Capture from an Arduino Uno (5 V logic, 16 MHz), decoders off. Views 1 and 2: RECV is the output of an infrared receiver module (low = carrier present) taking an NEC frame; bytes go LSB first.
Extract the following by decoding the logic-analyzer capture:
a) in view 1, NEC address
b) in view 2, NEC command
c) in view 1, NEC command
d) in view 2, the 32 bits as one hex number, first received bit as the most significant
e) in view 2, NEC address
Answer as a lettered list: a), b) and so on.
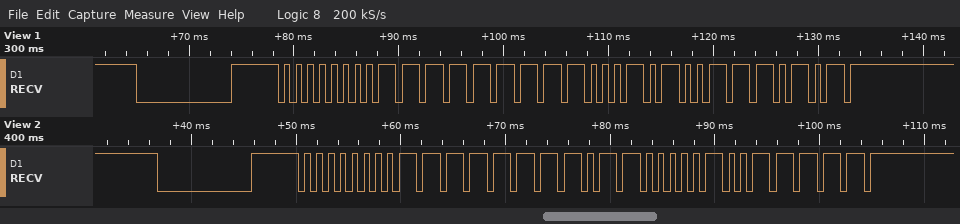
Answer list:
a) 0x00
b) 0x06
c) 0x51
d) 0x00FF609F
e) 0x00
